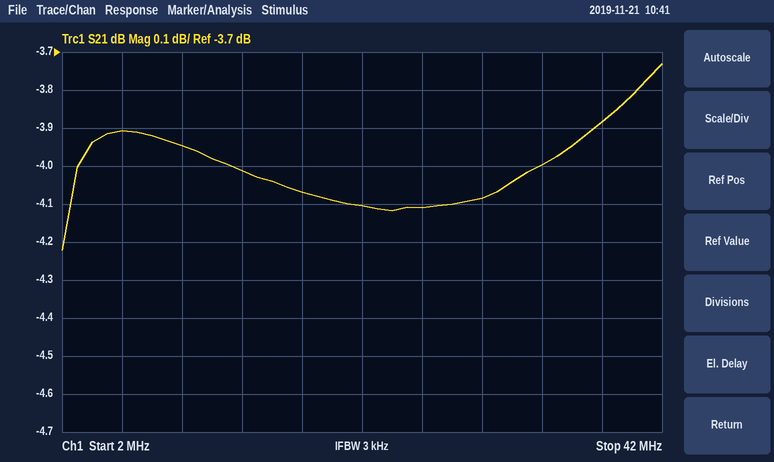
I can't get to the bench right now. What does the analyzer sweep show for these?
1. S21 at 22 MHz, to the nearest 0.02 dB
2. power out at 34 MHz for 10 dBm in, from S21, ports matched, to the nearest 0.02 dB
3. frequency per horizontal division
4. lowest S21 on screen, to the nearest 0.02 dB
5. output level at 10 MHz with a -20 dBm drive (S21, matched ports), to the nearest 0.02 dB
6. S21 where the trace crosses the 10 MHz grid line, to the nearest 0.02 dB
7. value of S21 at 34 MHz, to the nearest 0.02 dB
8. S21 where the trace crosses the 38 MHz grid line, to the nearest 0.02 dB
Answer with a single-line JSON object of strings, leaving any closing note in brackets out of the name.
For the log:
{"S21 at 22 MHz, to the nearest 0.02 dB": "-4.10 dB", "power out at 34 MHz for 10 dBm in, from S21, ports matched, to the nearest 0.02 dB": "6.00 dBm", "frequency per horizontal division": "4 MHz", "lowest S21 on screen, to the nearest 0.02 dB": "-4.22 dB", "output level at 10 MHz with a -20 dBm drive (S21, matched ports), to the nearest 0.02 dB": "-23.94 dBm", "S21 where the trace crosses the 10 MHz grid line, to the nearest 0.02 dB": "-3.94 dB", "value of S21 at 34 MHz, to the nearest 0.02 dB": "-4.00 dB", "S21 where the trace crosses the 38 MHz grid line, to the nearest 0.02 dB": "-3.88 dB"}
